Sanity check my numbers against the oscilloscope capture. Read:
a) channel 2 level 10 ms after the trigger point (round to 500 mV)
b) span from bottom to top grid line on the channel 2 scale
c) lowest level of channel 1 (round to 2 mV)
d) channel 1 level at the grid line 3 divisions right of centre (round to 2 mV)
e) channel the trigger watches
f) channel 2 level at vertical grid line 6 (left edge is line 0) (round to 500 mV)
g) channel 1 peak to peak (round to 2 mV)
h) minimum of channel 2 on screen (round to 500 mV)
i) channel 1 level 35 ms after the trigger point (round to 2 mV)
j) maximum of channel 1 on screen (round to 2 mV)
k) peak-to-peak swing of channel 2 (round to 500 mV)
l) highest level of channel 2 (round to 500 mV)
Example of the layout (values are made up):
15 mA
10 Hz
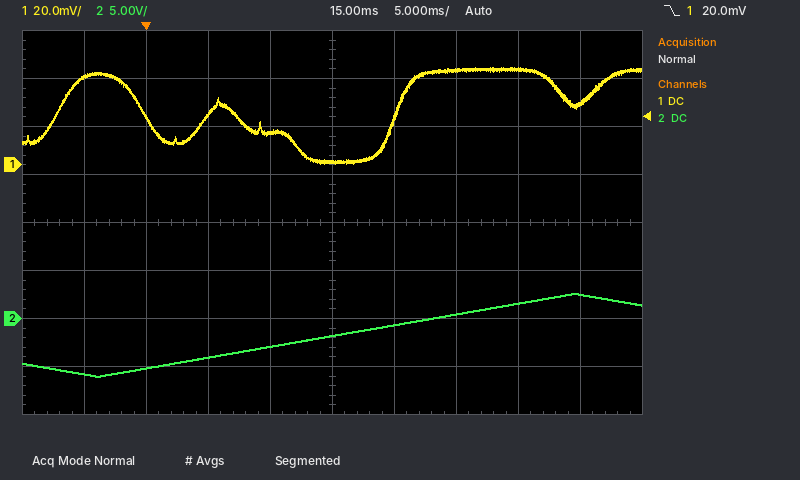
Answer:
-3.0 V
40 V
0 mV
40 mV
channel 1
-500 mV
40 mV
-6.0 V
26 mV
40 mV
8.5 V
2.5 V
